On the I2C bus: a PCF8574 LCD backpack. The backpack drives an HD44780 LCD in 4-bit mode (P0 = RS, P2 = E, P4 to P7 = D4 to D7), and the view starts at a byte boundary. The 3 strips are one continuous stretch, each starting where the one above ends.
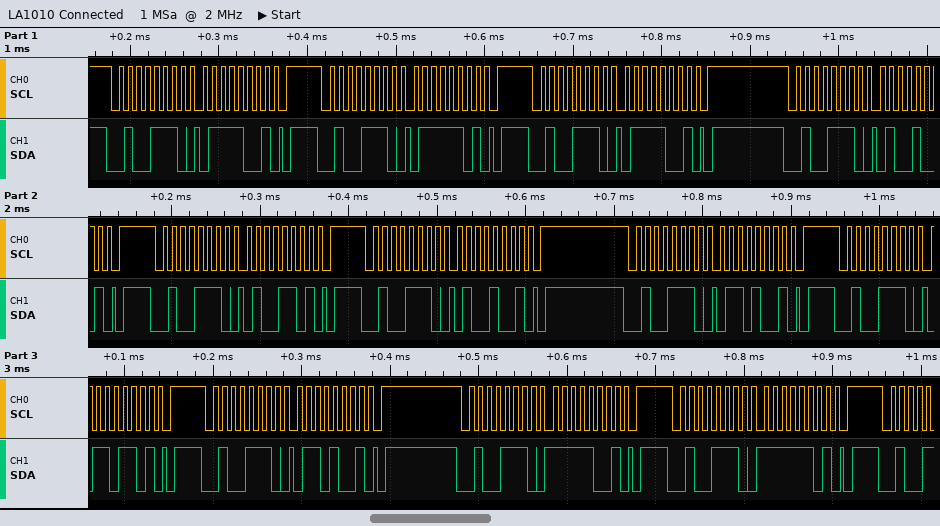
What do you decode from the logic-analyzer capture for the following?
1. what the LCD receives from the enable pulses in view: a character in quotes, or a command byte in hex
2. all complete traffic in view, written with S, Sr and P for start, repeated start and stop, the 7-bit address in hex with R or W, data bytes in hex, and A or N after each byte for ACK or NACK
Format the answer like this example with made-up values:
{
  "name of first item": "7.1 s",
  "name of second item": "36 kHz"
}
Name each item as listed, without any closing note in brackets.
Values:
{
  "what the LCD receives from the enable pulses in view: a character in quotes, or a command byte in hex": "'t'",
  "all complete traffic in view, written with S, Sr and P for start, repeated start and stop, the 7-bit address in hex with R or W, data bytes in hex, and A or N after each byte for ACK or NACK": "S 27W A 79 A P S 27W A 7D A P S 27W A 79 A P S 27W A 49 A P S 27W A 4D A P S 27W A 49 A P S 27W A 69 A P S 27W A 6D A P S 27W A 69 A P S 27W A F9 A P S 27W A FD A P"
}
